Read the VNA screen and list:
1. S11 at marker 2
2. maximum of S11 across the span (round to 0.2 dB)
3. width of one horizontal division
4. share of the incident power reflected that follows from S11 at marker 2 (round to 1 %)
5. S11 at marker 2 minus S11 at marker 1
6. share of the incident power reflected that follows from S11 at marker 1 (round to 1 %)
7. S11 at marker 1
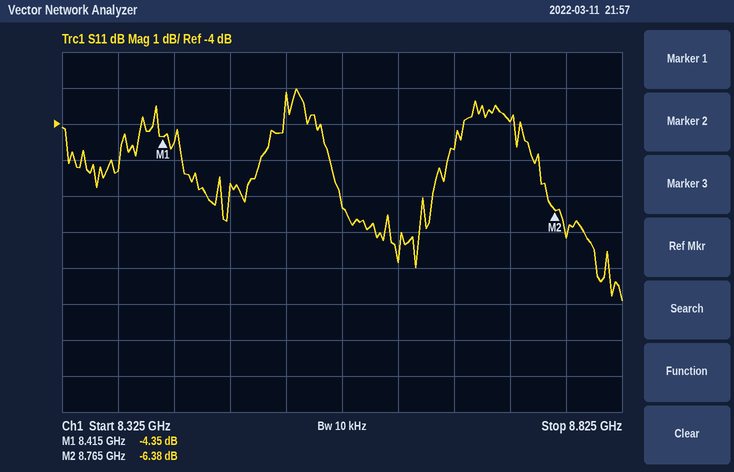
-6.38 dB
-3.0 dB
50 MHz
23 %
-2.03 dB
37 %
-4.35 dB
